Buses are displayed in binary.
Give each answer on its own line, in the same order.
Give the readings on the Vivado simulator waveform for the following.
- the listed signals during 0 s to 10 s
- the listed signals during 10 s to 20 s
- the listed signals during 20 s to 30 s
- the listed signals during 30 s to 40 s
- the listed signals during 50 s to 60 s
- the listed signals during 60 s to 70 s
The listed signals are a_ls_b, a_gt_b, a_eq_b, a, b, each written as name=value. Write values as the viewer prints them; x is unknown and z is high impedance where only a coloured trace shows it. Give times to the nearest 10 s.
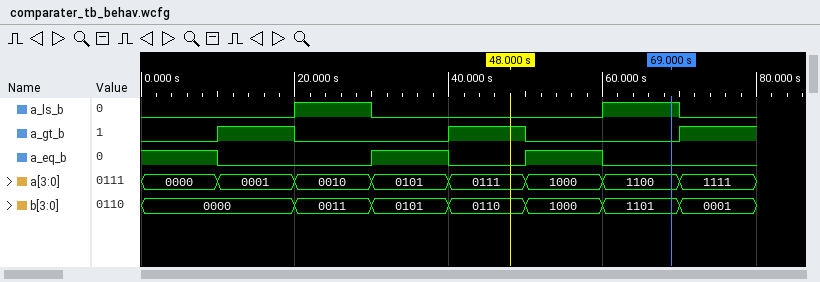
a_ls_b=0, a_gt_b=0, a_eq_b=1, a=0000, b=0000
a_ls_b=0, a_gt_b=1, a_eq_b=0, a=0001, b=0000
a_ls_b=1, a_gt_b=0, a_eq_b=0, a=0010, b=0011
a_ls_b=0, a_gt_b=0, a_eq_b=1, a=0101, b=0101
a_ls_b=0, a_gt_b=0, a_eq_b=1, a=1000, b=1000
a_ls_b=1, a_gt_b=0, a_eq_b=0, a=1100, b=1101
